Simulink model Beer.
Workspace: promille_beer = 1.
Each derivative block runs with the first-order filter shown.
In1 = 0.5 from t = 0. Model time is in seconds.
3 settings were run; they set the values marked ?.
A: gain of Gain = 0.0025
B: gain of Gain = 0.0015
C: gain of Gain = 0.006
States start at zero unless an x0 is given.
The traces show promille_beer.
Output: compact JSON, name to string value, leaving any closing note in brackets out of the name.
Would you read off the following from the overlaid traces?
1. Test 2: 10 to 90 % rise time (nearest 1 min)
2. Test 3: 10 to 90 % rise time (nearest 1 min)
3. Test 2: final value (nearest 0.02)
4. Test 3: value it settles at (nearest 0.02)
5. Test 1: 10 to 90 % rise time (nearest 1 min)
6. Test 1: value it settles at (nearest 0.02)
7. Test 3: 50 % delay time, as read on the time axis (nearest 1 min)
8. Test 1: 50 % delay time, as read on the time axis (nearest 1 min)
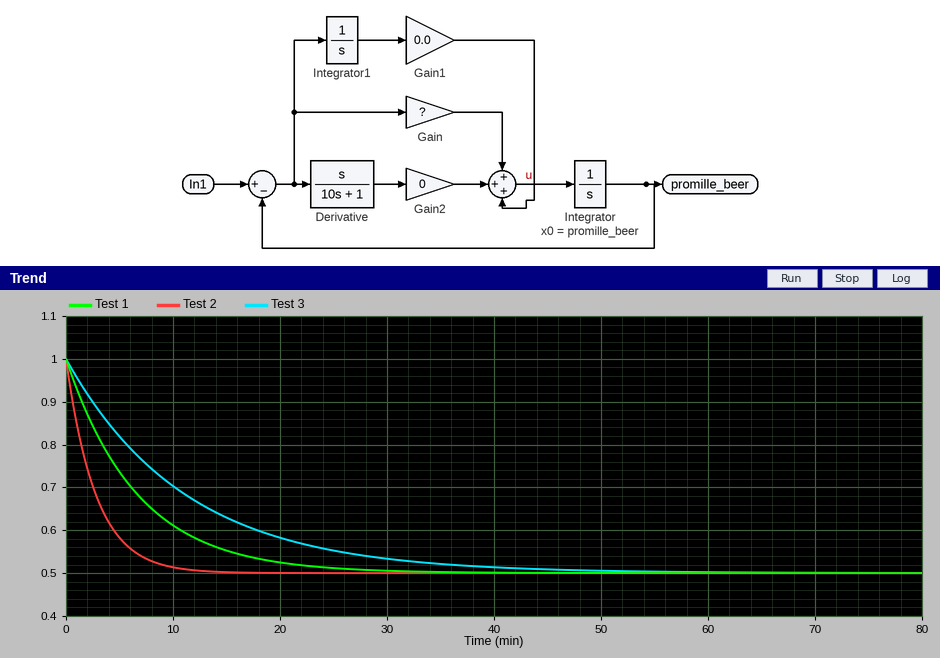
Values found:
{"Test 2: 10 to 90 % rise time": "6 min", "Test 3: 10 to 90 % rise time": "24 min", "Test 2: final value": "0.50", "Test 3: value it settles at": "0.50", "Test 1: 10 to 90 % rise time": "15 min", "Test 1: value it settles at": "0.50", "Test 3: 50 % delay time, as read on the time axis": "8 min", "Test 1: 50 % delay time, as read on the time axis": "5 min"}
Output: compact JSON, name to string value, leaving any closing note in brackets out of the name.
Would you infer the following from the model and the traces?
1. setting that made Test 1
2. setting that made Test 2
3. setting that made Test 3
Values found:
{"setting that made Test 1": "A", "setting that made Test 2": "C", "setting that made Test 3": "B"}
